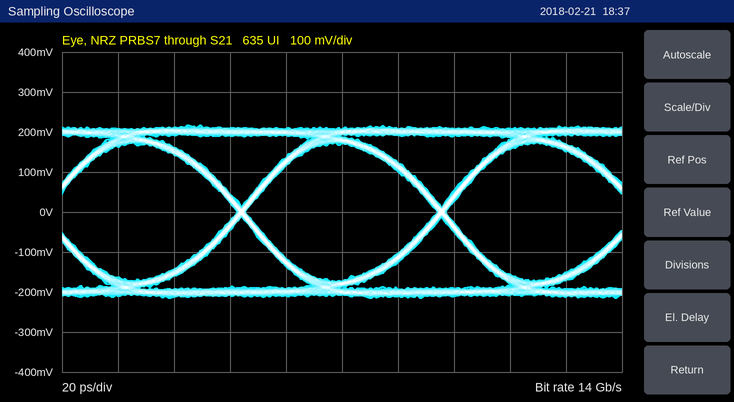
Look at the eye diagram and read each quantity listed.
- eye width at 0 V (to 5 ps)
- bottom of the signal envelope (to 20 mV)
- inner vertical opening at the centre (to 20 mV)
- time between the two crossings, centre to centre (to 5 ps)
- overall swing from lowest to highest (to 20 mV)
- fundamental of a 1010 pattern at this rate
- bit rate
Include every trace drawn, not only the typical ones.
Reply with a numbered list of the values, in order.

1. 70 ps
2. -220 mV
3. 340 mV
4. 70 ps
5. 440 mV
6. 7 GHz
7. 14 Gb/s
